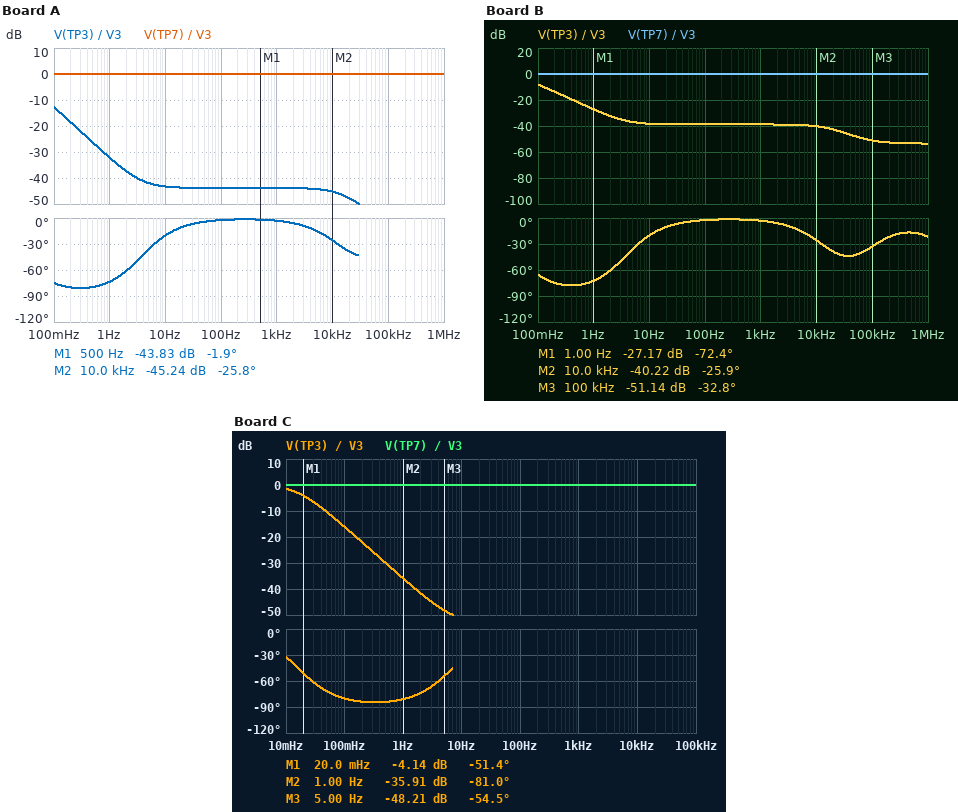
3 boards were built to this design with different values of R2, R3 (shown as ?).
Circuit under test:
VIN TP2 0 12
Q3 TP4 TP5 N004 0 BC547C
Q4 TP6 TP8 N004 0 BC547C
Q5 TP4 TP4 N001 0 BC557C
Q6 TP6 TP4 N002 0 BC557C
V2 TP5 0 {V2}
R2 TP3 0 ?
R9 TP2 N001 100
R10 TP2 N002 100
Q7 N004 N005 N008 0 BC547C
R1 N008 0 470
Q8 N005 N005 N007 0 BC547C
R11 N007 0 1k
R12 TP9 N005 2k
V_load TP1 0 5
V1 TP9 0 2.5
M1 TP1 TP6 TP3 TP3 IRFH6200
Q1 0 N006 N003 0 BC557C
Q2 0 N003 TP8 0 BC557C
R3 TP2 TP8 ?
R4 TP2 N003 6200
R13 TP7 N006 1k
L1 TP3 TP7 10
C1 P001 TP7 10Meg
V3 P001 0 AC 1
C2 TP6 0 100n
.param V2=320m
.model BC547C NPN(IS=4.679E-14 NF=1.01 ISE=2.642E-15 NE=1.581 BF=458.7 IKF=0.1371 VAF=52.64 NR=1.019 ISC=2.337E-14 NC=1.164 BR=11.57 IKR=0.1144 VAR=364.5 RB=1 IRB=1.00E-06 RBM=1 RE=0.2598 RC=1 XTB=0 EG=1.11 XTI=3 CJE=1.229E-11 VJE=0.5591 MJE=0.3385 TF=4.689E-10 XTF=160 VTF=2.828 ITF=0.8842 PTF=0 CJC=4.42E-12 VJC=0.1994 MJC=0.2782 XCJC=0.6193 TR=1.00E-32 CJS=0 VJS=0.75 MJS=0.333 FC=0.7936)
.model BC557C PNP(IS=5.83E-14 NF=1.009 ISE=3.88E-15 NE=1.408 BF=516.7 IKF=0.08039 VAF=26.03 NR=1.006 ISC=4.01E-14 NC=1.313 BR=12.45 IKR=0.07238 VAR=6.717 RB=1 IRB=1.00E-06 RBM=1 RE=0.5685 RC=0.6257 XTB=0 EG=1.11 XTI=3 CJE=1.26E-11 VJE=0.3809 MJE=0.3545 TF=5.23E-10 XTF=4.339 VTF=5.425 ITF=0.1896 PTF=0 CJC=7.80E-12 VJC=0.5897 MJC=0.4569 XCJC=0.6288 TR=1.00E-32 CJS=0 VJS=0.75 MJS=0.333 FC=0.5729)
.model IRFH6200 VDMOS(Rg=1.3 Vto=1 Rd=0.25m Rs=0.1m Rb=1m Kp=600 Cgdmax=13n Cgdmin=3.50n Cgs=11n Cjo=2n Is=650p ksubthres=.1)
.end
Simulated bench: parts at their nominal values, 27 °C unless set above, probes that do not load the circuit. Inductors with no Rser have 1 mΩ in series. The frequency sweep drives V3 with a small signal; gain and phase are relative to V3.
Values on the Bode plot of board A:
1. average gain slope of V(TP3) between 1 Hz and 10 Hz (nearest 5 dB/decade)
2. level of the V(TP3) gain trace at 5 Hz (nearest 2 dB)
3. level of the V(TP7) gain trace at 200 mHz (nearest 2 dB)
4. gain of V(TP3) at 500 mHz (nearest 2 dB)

-10 dB/decade
-42 dB
0 dB
-26 dB
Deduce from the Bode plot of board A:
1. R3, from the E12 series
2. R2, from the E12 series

8.2 kΩ
1.5 Ω
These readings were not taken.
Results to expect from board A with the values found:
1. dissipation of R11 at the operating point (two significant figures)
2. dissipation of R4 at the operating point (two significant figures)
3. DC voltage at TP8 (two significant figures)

310 µW
21 mW
1.2 V
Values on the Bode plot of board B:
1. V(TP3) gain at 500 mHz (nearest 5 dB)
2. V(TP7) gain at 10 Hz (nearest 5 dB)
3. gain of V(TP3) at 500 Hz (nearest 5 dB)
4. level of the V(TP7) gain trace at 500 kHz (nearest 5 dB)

-20 dB
0 dB
-40 dB
0 dB
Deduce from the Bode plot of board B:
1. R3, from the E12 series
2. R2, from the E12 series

8.2 kΩ
2.7 Ω
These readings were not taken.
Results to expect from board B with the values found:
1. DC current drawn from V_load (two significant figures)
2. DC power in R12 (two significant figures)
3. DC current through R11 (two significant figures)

290 µA
890 µW
560 µA
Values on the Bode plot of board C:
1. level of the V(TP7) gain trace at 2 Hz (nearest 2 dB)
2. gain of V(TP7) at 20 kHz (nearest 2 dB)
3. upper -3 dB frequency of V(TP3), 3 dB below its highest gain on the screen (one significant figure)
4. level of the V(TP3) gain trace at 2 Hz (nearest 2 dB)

0 dB
0 dB
20 mHz
-42 dB
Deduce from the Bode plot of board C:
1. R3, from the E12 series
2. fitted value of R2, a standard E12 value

10 kΩ
1 Ω
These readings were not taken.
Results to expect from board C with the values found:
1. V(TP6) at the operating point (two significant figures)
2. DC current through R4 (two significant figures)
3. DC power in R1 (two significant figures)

520 mV
1.8 mA
550 µW
